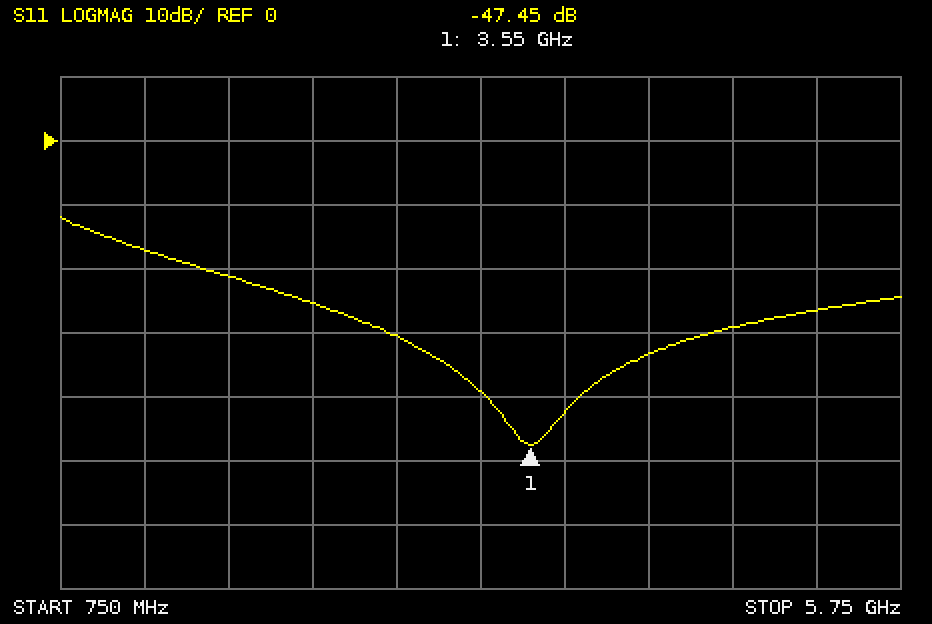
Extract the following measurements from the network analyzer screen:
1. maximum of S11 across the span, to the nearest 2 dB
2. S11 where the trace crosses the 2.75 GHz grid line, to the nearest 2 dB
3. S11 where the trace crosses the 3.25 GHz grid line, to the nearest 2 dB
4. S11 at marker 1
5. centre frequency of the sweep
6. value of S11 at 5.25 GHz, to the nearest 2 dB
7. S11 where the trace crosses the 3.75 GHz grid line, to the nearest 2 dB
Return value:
-12 dB
-30 dB
-40 dB
-47.45 dB
3.25 GHz
-26 dB
-42 dB
